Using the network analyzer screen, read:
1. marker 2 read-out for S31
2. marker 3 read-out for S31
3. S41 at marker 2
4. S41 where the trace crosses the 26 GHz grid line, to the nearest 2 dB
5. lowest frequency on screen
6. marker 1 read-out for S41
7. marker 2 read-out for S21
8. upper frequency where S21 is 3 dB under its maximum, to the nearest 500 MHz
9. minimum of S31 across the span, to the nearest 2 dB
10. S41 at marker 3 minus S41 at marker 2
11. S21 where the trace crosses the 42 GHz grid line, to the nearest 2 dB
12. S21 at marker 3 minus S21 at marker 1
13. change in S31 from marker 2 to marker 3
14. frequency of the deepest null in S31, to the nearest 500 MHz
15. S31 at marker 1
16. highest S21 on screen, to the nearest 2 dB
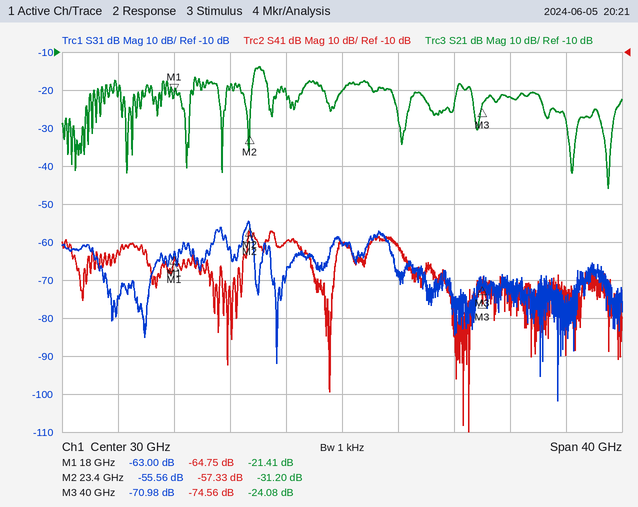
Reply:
-55.56 dB
-70.98 dB
-57.33 dB
-60 dB
10 GHz
-64.75 dB
-31.20 dB
24.5 GHz
-102 dB
-17.23 dB
-22 dB
-2.67 dB
-15.42 dB
45.5 GHz
-63.00 dB
-14 dB
